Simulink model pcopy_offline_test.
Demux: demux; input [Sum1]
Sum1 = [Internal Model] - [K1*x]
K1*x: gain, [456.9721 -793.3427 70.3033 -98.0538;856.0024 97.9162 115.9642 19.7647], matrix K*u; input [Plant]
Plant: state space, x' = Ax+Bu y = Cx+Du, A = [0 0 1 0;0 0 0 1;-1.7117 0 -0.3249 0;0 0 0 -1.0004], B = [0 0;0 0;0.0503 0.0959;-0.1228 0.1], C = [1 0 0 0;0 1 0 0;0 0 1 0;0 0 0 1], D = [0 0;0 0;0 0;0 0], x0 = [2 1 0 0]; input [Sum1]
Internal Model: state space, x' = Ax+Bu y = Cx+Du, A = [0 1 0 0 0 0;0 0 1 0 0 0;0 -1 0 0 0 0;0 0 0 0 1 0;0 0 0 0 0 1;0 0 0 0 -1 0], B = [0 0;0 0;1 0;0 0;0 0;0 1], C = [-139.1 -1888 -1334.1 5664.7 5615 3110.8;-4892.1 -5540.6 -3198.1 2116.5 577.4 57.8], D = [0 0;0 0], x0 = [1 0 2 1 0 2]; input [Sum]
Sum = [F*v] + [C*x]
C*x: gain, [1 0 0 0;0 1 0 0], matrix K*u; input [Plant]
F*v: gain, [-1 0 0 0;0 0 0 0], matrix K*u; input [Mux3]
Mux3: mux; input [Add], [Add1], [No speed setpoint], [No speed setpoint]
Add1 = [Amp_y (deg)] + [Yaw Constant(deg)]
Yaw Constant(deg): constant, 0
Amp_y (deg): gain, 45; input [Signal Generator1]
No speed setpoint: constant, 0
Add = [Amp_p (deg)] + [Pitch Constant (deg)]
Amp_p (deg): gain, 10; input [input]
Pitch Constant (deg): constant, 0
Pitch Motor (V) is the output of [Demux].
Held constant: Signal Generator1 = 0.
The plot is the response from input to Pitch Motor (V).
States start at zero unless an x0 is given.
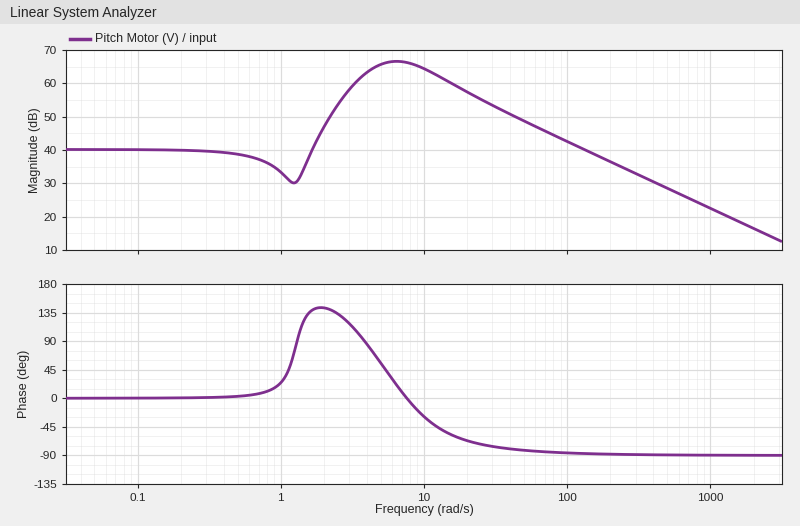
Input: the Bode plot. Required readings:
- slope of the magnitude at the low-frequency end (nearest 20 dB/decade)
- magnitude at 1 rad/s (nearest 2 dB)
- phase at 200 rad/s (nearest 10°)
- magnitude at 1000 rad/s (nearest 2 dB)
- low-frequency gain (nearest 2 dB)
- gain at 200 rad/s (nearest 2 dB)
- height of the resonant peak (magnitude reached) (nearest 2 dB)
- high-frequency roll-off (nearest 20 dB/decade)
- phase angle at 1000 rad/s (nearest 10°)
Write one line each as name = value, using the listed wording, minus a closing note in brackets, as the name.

slope of the magnitude at the low-frequency end = 0 dB/decade
magnitude at 1 rad/s = 34 dB
phase at 200 rad/s = -90°
magnitude at 1000 rad/s = 22 dB
low-frequency gain = 40 dB
gain at 200 rad/s = 36 dB
height of the resonant peak (magnitude reached) = 66 dB
high-frequency roll-off = -20 dB/decade
phase angle at 1000 rad/s = -90°
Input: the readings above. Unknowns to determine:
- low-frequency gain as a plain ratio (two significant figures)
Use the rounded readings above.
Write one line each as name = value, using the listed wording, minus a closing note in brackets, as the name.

low-frequency gain as a plain ratio = 100
